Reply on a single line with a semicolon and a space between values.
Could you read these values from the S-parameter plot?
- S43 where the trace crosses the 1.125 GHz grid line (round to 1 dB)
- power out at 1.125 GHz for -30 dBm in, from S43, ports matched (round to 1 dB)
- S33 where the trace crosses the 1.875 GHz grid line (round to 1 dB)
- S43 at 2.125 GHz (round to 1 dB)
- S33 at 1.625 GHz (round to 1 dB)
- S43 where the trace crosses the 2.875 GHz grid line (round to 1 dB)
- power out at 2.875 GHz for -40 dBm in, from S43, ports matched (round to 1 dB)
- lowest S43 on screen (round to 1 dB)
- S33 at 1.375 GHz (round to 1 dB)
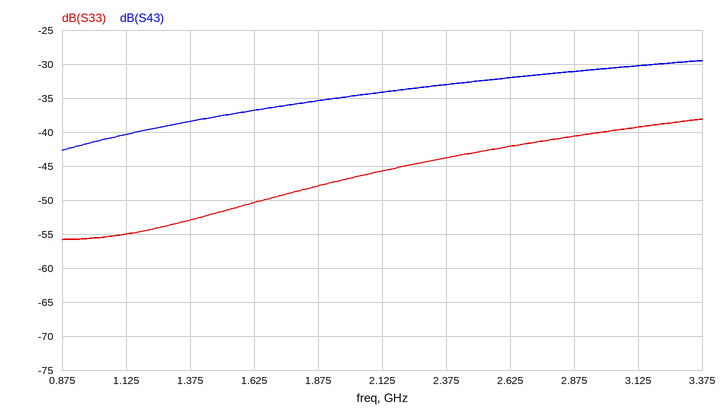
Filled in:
-40 dB; -70 dBm; -48 dB; -34 dB; -50 dB; -31 dB; -71 dBm; -43 dB; -53 dB
